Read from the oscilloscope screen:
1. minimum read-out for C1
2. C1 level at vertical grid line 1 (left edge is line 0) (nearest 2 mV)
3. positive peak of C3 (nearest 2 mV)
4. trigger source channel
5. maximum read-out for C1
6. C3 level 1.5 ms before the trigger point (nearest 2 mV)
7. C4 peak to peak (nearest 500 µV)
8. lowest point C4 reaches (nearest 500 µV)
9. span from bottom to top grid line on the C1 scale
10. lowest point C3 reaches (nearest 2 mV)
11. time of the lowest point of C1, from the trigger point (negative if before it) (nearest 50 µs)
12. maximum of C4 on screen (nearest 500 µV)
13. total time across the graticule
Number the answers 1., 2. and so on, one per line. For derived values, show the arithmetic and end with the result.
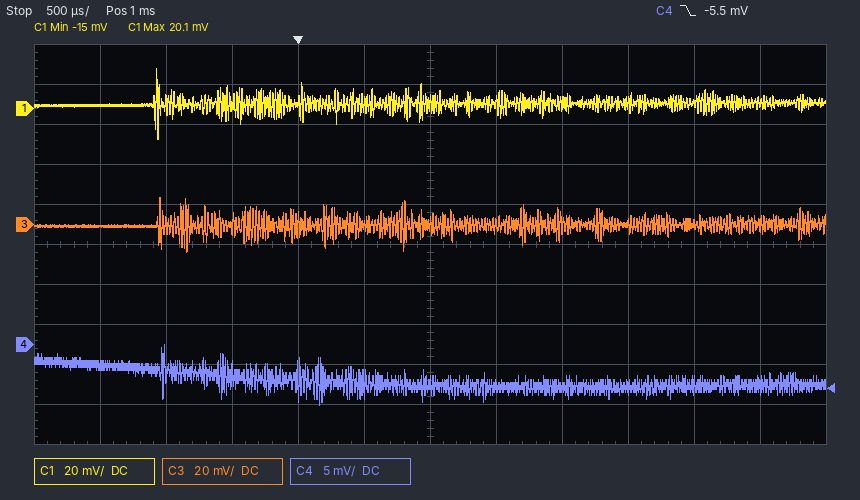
1. -15 mV
2. 2 mV
3. 14 mV
4. C4
5. 20.1 mV
6. 0 mV
7. 0.0 mV − (-7.5 mV) = 7.5 mV
8. -7.5 mV
9. 200 mV
10. -14 mV
11. -1.05 ms
12. 0.0 mV
13. 6 ms
